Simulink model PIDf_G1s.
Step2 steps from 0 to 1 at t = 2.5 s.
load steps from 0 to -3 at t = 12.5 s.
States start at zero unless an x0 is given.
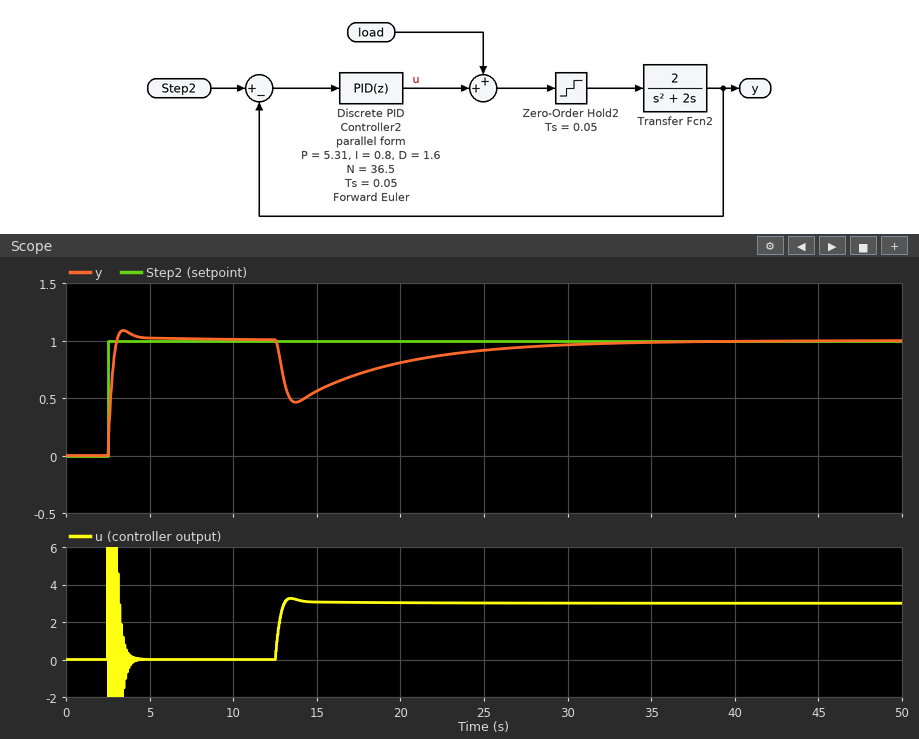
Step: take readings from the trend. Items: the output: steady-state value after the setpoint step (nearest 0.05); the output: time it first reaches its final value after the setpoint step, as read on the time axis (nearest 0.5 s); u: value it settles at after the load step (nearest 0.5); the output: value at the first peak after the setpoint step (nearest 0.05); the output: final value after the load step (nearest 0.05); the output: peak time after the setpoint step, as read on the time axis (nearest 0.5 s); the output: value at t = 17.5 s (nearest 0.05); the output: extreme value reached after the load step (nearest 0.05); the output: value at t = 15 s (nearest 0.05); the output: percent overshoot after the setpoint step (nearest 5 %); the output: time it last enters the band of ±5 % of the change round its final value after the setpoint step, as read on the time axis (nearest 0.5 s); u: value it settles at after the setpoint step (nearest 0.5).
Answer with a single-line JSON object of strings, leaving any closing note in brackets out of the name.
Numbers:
{"the output: steady-state value after the setpoint step": "1.00", "the output: time it first reaches its final value after the setpoint step, as read on the time axis": "3.0 s", "u: value it settles at after the load step": "3.0", "the output: value at the first peak after the setpoint step": "1.10", "the output: final value after the load step": "1.00", "the output: peak time after the setpoint step, as read on the time axis": "3.5 s", "the output: value at t = 17.5 s": "0.70", "the output: extreme value reached after the load step": "0.45", "the output: value at t = 15 s": "0.55", "the output: percent overshoot after the setpoint step": "10 %", "the output: time it last enters the band of ±5 % of the change round its final value after the setpoint step, as read on the time axis": "4.0 s", "u: value it settles at after the setpoint step": "0.0"}
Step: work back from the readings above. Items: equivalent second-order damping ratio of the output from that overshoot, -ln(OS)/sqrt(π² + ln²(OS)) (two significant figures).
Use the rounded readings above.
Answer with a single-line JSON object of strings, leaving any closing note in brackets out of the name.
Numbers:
{"equivalent second-order damping ratio of the output from that overshoot, -ln(OS)/sqrt(π² + ln²(OS))": "0.59"}
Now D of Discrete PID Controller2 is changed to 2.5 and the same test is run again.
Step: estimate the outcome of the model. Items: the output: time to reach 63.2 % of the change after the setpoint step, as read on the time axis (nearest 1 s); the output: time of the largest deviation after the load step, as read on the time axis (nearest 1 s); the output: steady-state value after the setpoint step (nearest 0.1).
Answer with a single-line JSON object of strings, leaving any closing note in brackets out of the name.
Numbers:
{"the output: time to reach 63.2 % of the change after the setpoint step, as read on the time axis": "3 s", "the output: time of the largest deviation after the load step, as read on the time axis": "14 s", "the output: steady-state value after the setpoint step": "1.0"}
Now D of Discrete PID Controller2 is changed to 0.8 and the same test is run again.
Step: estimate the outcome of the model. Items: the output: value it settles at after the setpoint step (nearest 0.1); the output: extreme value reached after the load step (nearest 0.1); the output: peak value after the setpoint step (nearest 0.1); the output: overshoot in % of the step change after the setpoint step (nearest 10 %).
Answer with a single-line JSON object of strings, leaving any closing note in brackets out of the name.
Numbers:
{"the output: value it settles at after the setpoint step": "1.0", "the output: extreme value reached after the load step": "0.4", "the output: peak value after the setpoint step": "1.2", "the output: overshoot in % of the step change after the setpoint step": "20 %"}
